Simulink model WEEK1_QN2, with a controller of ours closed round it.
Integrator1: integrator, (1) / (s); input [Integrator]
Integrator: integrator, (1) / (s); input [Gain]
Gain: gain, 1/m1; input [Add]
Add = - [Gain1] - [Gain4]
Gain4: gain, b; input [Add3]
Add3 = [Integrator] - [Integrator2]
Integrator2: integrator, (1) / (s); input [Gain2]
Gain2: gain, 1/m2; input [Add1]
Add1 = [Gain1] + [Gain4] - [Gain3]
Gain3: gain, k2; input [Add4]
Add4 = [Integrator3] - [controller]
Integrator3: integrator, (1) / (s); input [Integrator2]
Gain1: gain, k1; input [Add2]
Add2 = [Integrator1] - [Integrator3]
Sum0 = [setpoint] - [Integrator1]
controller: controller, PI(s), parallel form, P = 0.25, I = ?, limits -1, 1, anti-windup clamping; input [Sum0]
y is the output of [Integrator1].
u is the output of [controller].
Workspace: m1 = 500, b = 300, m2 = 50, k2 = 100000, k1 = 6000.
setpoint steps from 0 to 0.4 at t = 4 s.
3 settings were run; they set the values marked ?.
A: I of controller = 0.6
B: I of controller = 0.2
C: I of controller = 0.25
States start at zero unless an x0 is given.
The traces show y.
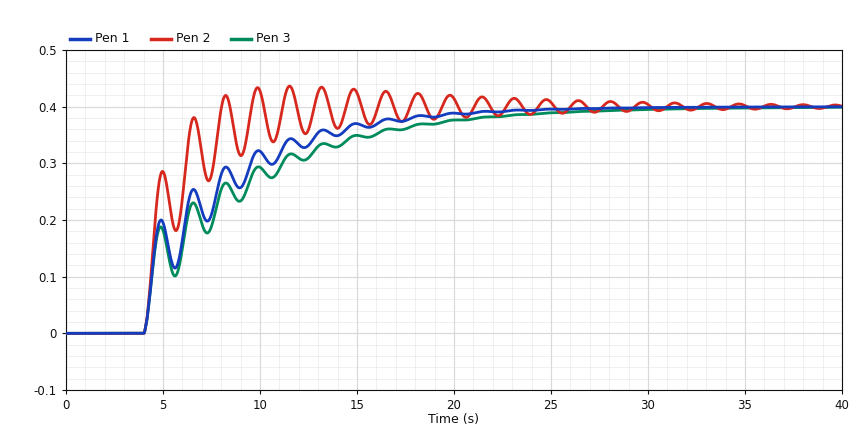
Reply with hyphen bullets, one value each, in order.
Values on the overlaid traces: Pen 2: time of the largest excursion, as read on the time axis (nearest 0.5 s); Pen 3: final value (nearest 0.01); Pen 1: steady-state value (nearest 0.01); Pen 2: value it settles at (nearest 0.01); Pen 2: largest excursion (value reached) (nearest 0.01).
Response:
- 11.5 s
- 0.40
- 0.40
- 0.40
- 0.44
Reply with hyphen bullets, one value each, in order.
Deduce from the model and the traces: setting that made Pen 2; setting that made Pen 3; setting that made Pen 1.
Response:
- A
- B
- C
